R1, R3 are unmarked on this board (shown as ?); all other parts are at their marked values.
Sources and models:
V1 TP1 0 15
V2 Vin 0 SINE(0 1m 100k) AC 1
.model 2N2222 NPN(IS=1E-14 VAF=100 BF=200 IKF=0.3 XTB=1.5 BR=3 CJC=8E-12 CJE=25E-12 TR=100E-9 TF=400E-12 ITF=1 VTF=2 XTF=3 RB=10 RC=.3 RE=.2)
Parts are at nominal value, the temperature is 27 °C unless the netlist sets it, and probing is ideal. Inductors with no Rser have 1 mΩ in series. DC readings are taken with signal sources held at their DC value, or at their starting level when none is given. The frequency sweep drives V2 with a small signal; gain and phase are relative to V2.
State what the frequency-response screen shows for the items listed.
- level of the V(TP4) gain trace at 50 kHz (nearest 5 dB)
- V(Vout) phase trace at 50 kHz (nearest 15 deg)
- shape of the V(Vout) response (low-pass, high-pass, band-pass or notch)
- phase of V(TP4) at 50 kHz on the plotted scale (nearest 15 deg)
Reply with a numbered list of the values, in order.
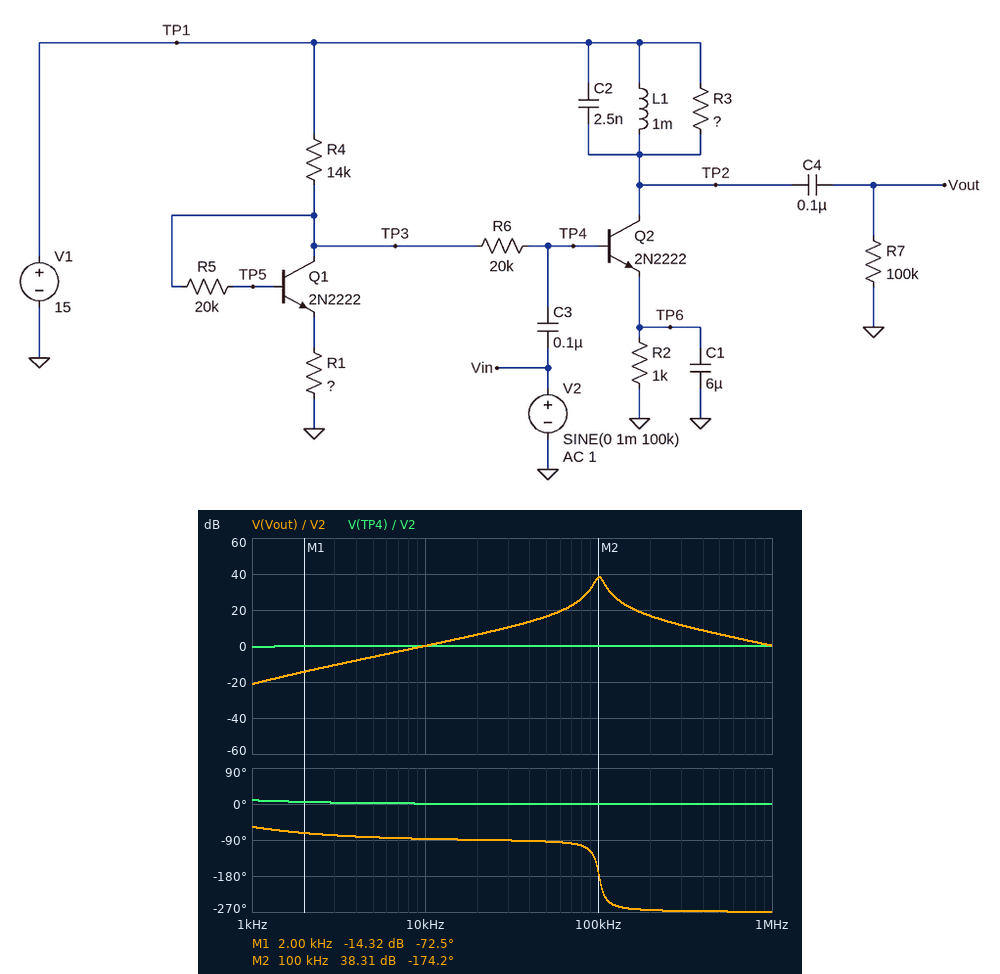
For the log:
1. 0 dB
2. -90 deg
3. band-pass
4. 0 deg
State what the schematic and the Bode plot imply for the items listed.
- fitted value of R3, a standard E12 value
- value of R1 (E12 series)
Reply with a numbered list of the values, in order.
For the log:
1. 5.6 kΩ
2. 330 Ω
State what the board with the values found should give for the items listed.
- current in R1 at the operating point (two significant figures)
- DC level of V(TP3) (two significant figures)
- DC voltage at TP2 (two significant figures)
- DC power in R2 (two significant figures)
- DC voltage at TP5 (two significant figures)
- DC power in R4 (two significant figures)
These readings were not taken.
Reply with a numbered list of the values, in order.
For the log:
1. 990 µA
2. 1.1 V
3. 15 V
4. 170 µW
5. 980 mV
6. 14 mW
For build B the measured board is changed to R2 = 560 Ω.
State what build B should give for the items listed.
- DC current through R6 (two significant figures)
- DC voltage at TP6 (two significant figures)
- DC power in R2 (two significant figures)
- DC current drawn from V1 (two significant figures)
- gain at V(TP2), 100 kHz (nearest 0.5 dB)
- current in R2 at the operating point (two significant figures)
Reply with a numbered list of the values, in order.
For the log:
1. 3.0 µA
2. 380 mV
3. 260 µW
4. 1.7 mA
5. 42.5 dB
6. 680 µA
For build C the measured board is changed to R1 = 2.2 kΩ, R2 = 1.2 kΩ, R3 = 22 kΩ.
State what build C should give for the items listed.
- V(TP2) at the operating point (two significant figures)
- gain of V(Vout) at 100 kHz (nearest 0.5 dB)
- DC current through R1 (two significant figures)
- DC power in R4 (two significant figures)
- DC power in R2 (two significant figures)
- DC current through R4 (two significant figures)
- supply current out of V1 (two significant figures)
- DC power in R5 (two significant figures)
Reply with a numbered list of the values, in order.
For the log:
1. 15 V
2. 58.0 dB
3. 870 µA
4. 11 mW
5. 2.9 mW
6. 880 µA
7. 2.4 mA
8. 380 nW
